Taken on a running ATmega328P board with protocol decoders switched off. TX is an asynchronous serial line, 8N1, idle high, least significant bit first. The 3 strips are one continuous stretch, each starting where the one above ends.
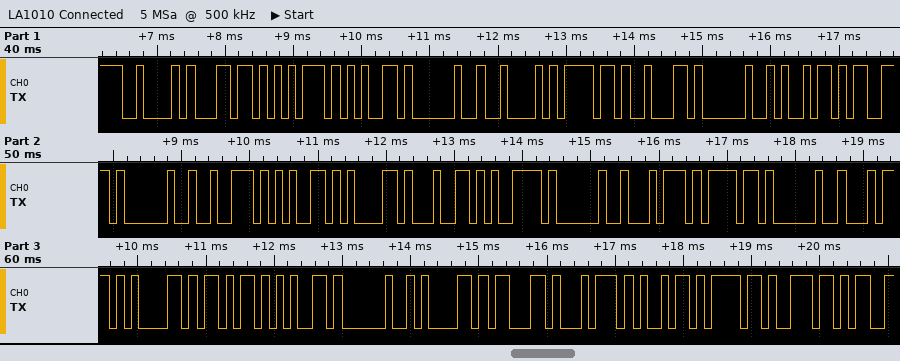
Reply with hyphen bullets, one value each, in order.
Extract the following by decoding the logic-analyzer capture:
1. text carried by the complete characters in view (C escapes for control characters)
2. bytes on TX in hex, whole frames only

- "Blue Bob is ready to take action"
- 42 6C 75 65 20 42 6F 62 20 69 73 20 72 65 61 64 79 20 74 6F 20 74 61 6B 65 20 61 63 74 69 6F 6E
